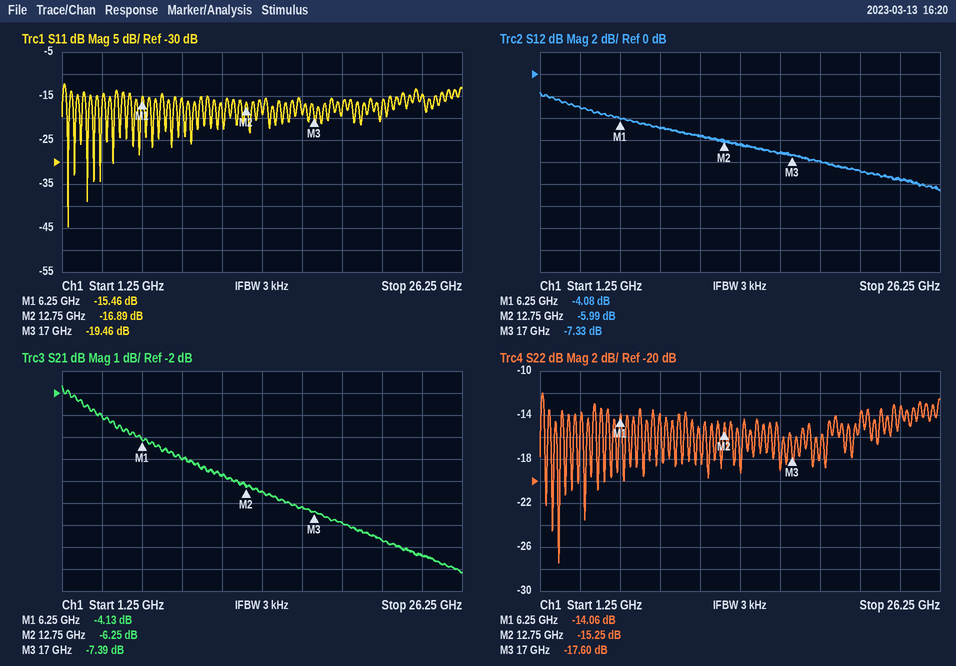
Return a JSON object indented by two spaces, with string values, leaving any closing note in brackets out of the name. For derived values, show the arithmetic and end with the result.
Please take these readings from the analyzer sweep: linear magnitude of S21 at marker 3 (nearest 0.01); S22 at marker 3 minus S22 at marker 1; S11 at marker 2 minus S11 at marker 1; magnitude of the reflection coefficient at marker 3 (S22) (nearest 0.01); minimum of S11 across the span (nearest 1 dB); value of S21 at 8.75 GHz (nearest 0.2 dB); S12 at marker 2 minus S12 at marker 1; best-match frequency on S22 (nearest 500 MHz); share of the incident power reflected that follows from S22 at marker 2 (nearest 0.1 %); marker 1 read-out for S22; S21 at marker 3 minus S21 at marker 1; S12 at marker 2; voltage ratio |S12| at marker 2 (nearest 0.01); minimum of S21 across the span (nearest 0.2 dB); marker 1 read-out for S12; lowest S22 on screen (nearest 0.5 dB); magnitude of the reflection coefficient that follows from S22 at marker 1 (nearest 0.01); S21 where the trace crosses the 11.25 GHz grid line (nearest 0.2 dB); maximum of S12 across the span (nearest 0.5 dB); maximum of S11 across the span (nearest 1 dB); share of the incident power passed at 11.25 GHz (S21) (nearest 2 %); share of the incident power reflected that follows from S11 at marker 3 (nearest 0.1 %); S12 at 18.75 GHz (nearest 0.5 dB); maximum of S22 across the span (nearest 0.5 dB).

{
  "linear magnitude of S21 at marker 3": "10^(-7.39/20) ≈ 0.43",
  "S22 at marker 3 minus S22 at marker 1": "-17.6 − (-14.06) = -3.54 dB",
  "S11 at marker 2 minus S11 at marker 1": "-16.89 − (-15.46) = -1.43 dB",
  "magnitude of the reflection coefficient at marker 3 (S22)": "10^(-17.6/20) ≈ 0.13",
  "minimum of S11 across the span": "-45 dB",
  "value of S21 at 8.75 GHz": "-5.0 dB",
  "S12 at marker 2 minus S12 at marker 1": "-5.99 − (-4.08) = -1.91 dB",
  "best-match frequency on S22": "2.5 GHz",
  "share of the incident power reflected that follows from S22 at marker 2": "10^(-15.25/10) ≈ 3.0 %",
  "marker 1 read-out for S22": "-14.06 dB",
  "S21 at marker 3 minus S21 at marker 1": "-7.39 − (-4.13) = -3.26 dB",
  "S12 at marker 2": "-5.99 dB",
  "voltage ratio |S12| at marker 2": "10^(-5.99/20) ≈ 0.50",
  "minimum of S21 across the span": "-10.2 dB",
  "marker 1 read-out for S12": "-4.08 dB",
  "lowest S22 on screen": "-27.5 dB",
  "magnitude of the reflection coefficient that follows from S22 at marker 1": "10^(-14.06/20) ≈ 0.20",
  "S21 where the trace crosses the 11.25 GHz grid line": "-5.8 dB",
  "maximum of S12 across the span": "-1.5 dB",
  "maximum of S11 across the span": "-12 dB",
  "share of the incident power passed at 11.25 GHz (S21)": "10^(-5.8/10) ≈ 26 %",
  "share of the incident power reflected that follows from S11 at marker 3": "10^(-19.46/10) ≈ 1.1 %",
  "S12 at 18.75 GHz": "-8.0 dB",
  "maximum of S22 across the span": "-12.0 dB"
}
